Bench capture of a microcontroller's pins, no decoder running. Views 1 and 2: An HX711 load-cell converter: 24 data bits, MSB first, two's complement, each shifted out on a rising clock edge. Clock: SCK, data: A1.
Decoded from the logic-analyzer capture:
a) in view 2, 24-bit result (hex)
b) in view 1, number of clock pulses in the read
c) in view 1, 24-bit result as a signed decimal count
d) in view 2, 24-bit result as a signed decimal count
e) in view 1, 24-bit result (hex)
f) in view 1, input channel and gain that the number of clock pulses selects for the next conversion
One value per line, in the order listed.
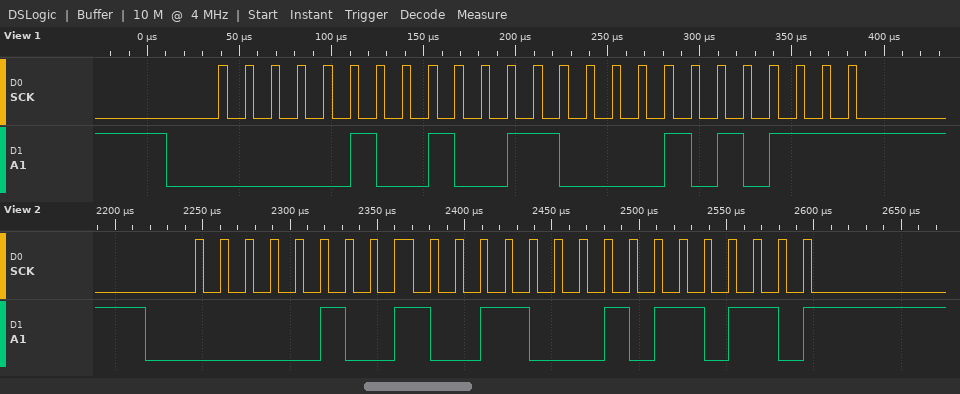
0x0498B6
25
301143
301238
0x049857
channel A, gain 128
